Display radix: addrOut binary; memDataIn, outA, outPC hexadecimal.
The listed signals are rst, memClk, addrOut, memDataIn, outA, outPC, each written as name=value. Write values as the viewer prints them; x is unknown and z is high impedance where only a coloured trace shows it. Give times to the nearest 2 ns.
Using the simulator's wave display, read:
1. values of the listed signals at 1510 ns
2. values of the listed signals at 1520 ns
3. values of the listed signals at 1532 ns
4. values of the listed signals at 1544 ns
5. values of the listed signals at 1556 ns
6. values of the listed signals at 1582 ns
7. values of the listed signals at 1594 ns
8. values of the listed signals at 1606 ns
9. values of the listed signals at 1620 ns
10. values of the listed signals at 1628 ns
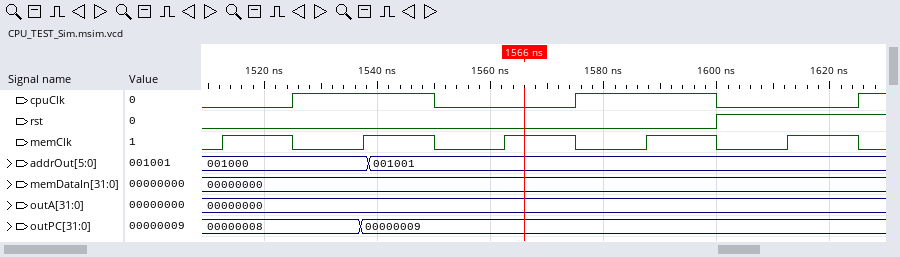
rst=0, memClk=0, addrOut=001000, memDataIn=00000000, outA=00000000, outPC=00000008
rst=0, memClk=1, addrOut=001000, memDataIn=00000000, outA=00000000, outPC=00000008
rst=0, memClk=0, addrOut=001000, memDataIn=00000000, outA=00000000, outPC=00000008
rst=0, memClk=1, addrOut=001001, memDataIn=00000000, outA=00000000, outPC=00000009
rst=0, memClk=0, addrOut=001001, memDataIn=00000000, outA=00000000, outPC=00000009
rst=0, memClk=0, addrOut=001001, memDataIn=00000000, outA=00000000, outPC=00000009
rst=0, memClk=1, addrOut=001001, memDataIn=00000000, outA=00000000, outPC=00000009
rst=1, memClk=0, addrOut=001001, memDataIn=00000000, outA=00000000, outPC=00000009
rst=1, memClk=1, addrOut=001001, memDataIn=00000000, outA=00000000, outPC=00000009
rst=1, memClk=0, addrOut=001001, memDataIn=00000000, outA=00000000, outPC=00000009
